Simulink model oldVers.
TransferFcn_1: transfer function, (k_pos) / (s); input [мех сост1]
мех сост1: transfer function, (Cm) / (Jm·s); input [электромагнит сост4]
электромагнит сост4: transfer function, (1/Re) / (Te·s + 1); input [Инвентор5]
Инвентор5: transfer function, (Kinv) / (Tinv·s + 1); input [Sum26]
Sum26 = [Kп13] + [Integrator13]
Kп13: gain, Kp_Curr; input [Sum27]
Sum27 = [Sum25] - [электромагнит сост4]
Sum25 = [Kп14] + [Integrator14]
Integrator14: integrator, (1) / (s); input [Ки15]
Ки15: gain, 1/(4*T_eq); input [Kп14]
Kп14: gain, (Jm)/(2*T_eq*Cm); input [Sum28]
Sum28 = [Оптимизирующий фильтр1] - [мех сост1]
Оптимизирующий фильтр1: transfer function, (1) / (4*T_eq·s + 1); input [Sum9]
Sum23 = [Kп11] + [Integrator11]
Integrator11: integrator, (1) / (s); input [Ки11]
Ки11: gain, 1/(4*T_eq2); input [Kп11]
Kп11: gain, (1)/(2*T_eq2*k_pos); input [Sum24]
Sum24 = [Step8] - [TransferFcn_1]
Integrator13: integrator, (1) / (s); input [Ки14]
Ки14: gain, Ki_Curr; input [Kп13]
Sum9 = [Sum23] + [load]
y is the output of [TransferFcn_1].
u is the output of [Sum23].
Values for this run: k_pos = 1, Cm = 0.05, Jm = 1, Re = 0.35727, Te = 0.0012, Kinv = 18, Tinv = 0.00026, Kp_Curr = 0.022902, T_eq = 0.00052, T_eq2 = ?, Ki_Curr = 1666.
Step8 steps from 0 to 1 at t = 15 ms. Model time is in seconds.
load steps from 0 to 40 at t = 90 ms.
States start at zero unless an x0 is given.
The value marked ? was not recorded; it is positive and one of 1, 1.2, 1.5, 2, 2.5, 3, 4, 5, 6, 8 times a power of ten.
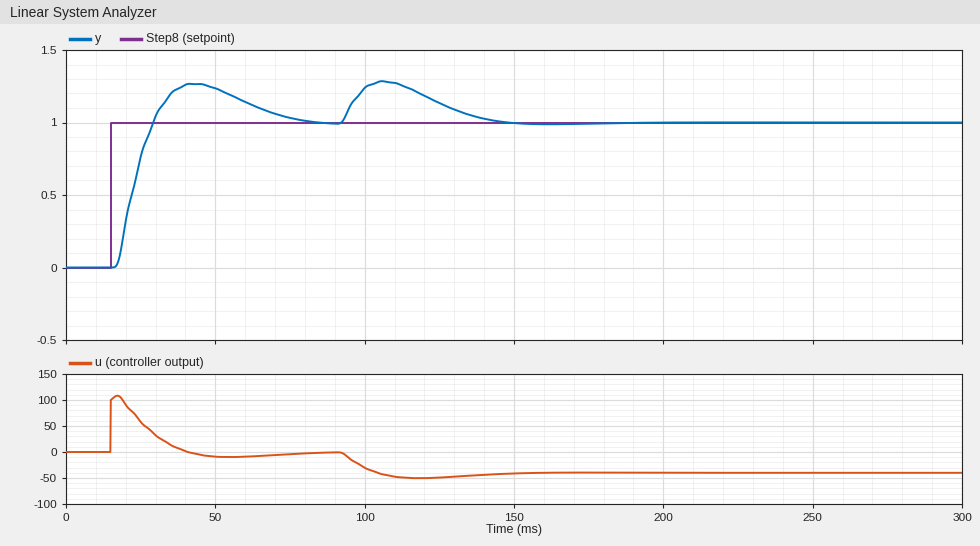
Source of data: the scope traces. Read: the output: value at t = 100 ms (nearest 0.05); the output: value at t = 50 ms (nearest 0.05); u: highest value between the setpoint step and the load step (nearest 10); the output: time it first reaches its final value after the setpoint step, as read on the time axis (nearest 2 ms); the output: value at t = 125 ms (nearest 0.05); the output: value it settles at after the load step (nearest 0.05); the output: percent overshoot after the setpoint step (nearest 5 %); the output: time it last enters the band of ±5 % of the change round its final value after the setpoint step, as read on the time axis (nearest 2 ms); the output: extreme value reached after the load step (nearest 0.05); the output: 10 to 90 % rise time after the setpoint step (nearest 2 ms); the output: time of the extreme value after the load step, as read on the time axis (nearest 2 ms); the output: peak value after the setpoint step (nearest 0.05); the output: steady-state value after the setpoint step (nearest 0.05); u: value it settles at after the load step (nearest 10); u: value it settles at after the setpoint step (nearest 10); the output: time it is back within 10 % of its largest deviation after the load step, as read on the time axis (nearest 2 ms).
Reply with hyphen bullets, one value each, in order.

- 1.25
- 1.25
- 110
- 30 ms
- 1.15
- 1.00
- 25 %
- 72 ms
- 1.30
- 10 ms
- 106 ms
- 1.25
- 1.00
- -40
- 0
- 140 ms
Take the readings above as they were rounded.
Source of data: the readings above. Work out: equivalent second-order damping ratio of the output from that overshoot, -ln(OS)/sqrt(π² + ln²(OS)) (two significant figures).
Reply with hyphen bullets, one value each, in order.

- 0.40
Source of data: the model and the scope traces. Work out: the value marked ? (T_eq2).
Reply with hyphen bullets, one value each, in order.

- 0.005
